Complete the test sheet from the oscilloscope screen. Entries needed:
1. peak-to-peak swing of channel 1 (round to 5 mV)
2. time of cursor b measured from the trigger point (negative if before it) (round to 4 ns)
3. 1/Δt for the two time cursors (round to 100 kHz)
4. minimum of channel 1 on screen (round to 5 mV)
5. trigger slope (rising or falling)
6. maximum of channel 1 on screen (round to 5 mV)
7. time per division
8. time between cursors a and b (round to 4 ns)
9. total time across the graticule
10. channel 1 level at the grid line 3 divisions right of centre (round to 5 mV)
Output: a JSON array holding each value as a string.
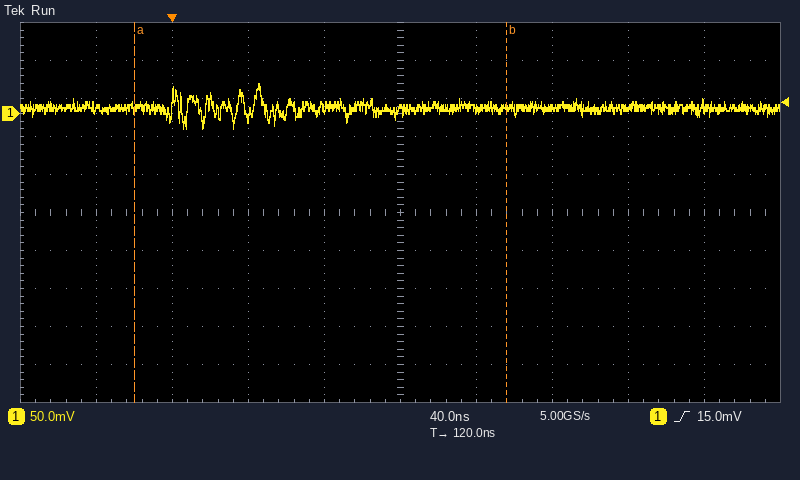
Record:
["60 mV", "+176 ns", "5.1 MHz", "-20 mV", "rising", "40 mV", "40 ns", "196 ns", "400 ns", "10 mV"]
